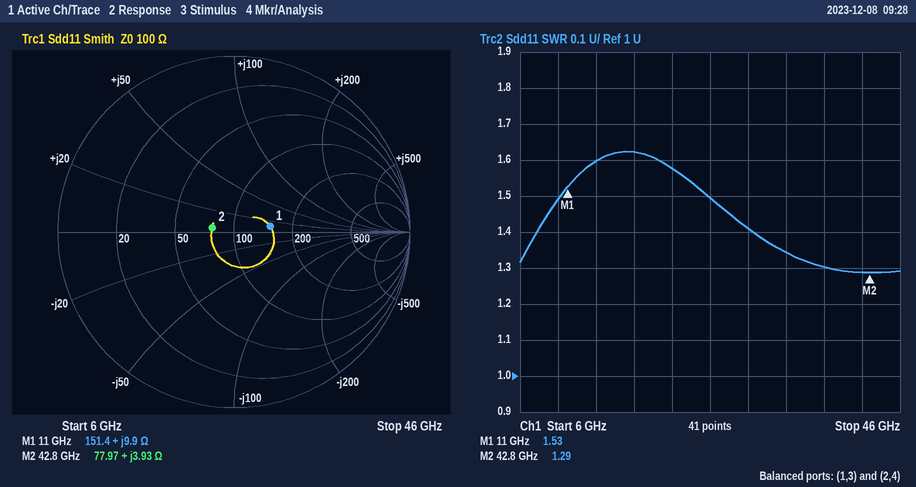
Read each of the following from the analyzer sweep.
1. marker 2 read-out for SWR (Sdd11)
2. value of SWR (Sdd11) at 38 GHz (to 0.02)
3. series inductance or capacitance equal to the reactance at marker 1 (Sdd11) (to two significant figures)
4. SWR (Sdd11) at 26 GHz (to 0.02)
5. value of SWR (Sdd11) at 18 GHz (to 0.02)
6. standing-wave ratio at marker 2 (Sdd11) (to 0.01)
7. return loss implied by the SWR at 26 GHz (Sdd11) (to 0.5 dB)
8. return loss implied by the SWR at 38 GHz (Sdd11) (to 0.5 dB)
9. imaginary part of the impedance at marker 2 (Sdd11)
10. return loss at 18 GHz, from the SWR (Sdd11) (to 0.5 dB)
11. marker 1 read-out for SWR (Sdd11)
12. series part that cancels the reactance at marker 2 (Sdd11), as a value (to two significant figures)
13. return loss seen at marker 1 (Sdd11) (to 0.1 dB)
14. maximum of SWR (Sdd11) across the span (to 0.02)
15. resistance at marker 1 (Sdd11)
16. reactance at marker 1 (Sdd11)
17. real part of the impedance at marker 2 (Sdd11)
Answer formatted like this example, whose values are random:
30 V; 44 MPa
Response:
1.29; 1.30; 140 pH; 1.50; 1.62; 1.29; 14.0 dB; 17.5 dB; +3.93 Ω; 12.5 dB; 1.53; 950 fF; 13.6 dB; 1.62; 151.4 Ω; +9.9 Ω; 77.97 Ω
